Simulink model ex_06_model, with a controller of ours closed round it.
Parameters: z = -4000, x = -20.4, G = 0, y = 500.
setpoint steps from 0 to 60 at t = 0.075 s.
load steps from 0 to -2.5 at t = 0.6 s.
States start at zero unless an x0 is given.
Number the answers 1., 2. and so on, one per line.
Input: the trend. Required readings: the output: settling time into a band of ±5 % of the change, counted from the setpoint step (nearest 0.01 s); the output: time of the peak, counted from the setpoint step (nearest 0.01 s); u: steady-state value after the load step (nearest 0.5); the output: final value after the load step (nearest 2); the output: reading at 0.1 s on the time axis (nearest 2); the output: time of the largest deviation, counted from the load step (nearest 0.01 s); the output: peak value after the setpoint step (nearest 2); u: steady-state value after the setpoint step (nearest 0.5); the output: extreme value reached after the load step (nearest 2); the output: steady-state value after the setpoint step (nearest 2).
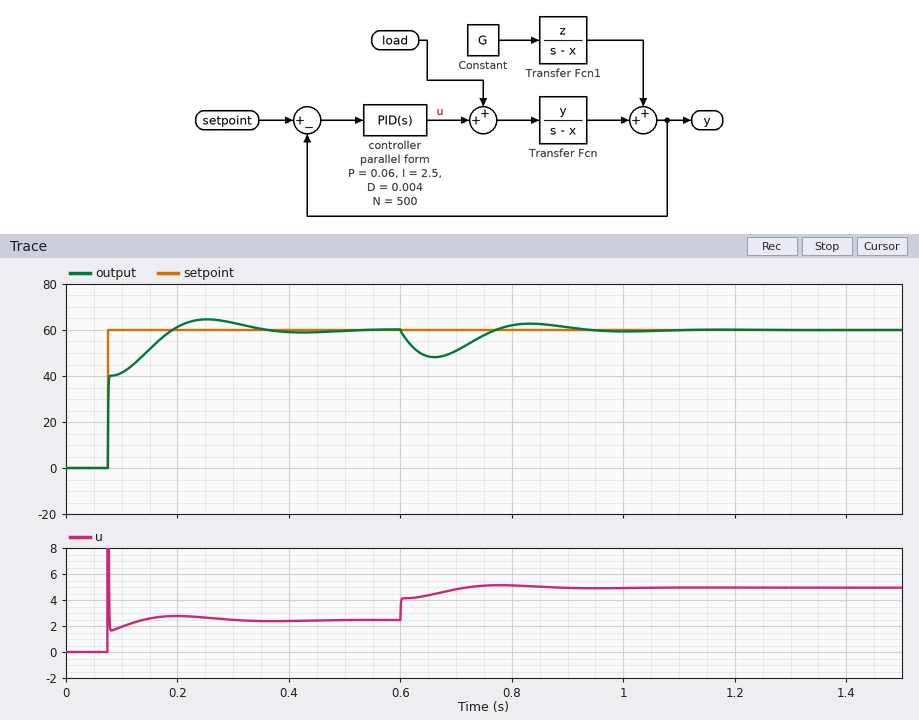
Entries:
1. 0.23 s
2. 0.18 s
3. 5.0
4. 60
5. 42
6. 0.06 s
7. 64
8. 2.5
9. 48
10. 60
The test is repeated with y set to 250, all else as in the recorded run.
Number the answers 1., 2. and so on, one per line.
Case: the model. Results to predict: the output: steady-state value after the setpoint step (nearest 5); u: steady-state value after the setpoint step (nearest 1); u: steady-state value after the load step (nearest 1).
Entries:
1. 60
2. 5
3. 7
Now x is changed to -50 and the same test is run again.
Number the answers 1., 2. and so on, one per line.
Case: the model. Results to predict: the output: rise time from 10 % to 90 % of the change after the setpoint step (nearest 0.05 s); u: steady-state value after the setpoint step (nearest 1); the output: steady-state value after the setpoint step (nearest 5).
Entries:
1. 0.15 s
2. 6
3. 60
